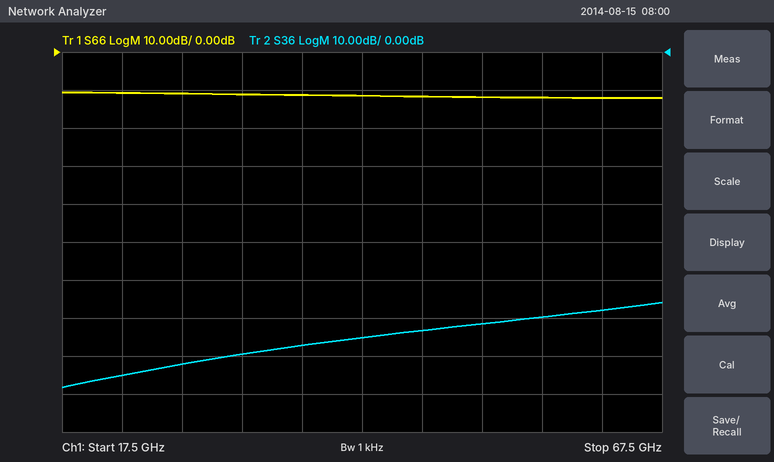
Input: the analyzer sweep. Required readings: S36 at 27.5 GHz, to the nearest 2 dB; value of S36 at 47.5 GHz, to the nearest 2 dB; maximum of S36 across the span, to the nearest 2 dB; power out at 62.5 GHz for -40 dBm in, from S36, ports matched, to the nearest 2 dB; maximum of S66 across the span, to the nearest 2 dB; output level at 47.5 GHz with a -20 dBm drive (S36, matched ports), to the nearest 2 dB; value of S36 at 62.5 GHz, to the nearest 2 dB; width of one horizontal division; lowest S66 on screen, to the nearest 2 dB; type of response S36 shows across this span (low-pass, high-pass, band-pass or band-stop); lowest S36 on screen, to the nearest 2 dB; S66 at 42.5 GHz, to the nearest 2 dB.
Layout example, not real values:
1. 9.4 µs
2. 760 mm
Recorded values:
1. -82 dB
2. -74 dB
3. -66 dB
4. -108 dBm
5. -10 dB
6. -94 dBm
7. -68 dB
8. 5 GHz
9. -12 dB
10. high-pass
11. -88 dB
12. -12 dB
